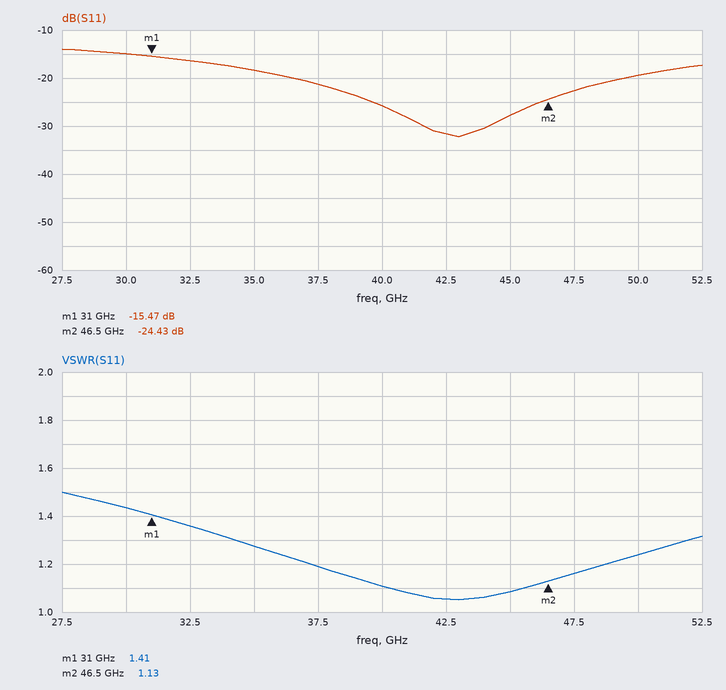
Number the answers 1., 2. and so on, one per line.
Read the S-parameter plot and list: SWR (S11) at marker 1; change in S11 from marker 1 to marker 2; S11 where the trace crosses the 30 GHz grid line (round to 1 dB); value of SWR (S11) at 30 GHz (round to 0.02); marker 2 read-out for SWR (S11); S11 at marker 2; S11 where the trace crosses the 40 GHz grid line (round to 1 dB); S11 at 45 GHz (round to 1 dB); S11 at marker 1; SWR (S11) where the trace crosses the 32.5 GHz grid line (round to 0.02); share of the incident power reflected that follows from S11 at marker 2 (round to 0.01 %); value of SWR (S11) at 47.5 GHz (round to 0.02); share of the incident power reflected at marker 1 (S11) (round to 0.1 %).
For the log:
1. 1.41
2. -8.96 dB
3. -15 dB
4. 1.44
5. 1.13
6. -24.43 dB
7. -26 dB
8. -28 dB
9. -15.47 dB
10. 1.36
11. 0.36 %
12. 1.16
13. 2.8 %
